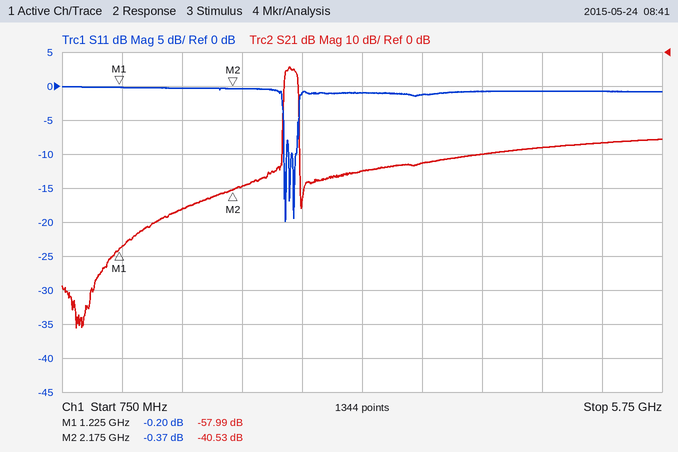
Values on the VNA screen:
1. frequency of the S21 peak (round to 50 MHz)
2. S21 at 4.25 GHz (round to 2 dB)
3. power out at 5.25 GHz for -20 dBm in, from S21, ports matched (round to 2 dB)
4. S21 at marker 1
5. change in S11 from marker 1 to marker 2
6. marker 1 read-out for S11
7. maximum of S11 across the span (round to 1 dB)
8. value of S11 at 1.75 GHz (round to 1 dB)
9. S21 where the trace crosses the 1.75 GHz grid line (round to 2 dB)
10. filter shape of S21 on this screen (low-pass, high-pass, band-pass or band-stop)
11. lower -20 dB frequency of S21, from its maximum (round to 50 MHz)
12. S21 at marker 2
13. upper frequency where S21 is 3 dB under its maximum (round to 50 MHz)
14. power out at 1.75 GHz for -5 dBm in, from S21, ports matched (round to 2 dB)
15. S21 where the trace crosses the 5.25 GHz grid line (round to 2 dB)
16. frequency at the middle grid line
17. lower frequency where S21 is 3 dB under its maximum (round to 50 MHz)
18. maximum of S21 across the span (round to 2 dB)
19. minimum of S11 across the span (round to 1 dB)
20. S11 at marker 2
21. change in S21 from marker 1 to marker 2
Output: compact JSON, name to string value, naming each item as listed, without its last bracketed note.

{"frequency of the S21 peak": "2.65 GHz", "S21 at 4.25 GHz": "-30 dB", "power out at 5.25 GHz for -20 dBm in, from S21, ports matched": "-46 dBm", "S21 at marker 1": "-57.99 dB", "change in S11 from marker 1 to marker 2": "-0.17 dB", "marker 1 read-out for S11": "-0.20 dB", "maximum of S11 across the span": "0 dB", "value of S11 at 1.75 GHz": "0 dB", "S21 where the trace crosses the 1.75 GHz grid line": "-46 dB", "filter shape of S21 on this screen": "band-pass", "lower -20 dB frequency of S21, from its maximum": "2.60 GHz", "S21 at marker 2": "-40.53 dB", "upper frequency where S21 is 3 dB under its maximum": "2.70 GHz", "power out at 1.75 GHz for -5 dBm in, from S21, ports matched": "-52 dBm", "S21 where the trace crosses the 5.25 GHz grid line": "-26 dB", "frequency at the middle grid line": "3.25 GHz", "lower frequency where S21 is 3 dB under its maximum": "2.60 GHz", "maximum of S21 across the span": "-4 dB", "minimum of S11 across the span": "-20 dB", "S11 at marker 2": "-0.37 dB", "change in S21 from marker 1 to marker 2": "17.46 dB"}
